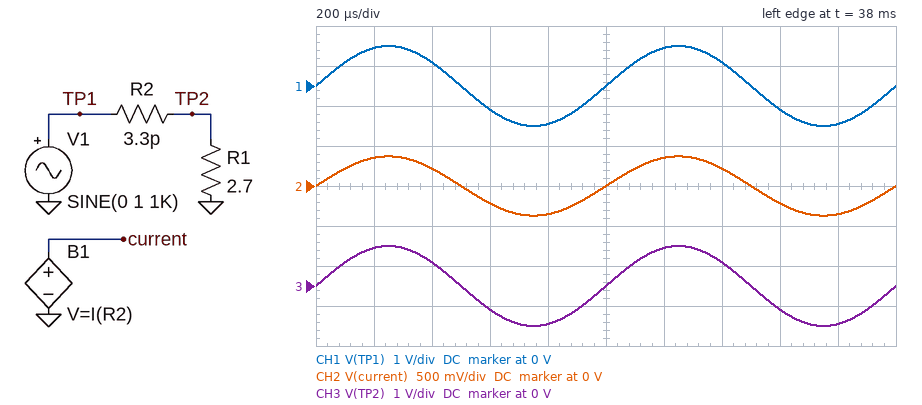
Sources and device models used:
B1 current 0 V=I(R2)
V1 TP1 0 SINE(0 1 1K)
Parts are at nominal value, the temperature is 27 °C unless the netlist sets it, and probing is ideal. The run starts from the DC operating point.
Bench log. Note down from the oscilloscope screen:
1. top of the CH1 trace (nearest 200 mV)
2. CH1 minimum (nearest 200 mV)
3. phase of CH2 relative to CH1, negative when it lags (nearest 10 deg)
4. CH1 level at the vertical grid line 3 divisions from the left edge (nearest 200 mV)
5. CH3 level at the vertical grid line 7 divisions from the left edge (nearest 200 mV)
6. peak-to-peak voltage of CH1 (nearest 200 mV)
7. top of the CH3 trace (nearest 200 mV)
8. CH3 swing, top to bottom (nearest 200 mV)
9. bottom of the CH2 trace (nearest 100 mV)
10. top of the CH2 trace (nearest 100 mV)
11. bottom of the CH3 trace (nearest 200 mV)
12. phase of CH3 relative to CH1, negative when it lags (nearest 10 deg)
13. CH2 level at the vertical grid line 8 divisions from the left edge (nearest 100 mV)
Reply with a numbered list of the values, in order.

1. 1.0 V
2. -1.0 V
3. 0 deg
4. -600 mV
5. 600 mV
6. 2.0 V
7. 1.0 V
8. 2.0 V
9. -400 mV
10. 400 mV
11. -1.0 V
12. 0 deg
13. -200 mV
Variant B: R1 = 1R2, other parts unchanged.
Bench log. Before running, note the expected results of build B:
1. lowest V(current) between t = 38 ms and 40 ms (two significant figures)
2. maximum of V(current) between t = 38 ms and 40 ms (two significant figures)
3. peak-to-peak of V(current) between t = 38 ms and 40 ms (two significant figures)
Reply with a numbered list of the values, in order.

1. -830 mV
2. 830 mV
3. 1.7 V
